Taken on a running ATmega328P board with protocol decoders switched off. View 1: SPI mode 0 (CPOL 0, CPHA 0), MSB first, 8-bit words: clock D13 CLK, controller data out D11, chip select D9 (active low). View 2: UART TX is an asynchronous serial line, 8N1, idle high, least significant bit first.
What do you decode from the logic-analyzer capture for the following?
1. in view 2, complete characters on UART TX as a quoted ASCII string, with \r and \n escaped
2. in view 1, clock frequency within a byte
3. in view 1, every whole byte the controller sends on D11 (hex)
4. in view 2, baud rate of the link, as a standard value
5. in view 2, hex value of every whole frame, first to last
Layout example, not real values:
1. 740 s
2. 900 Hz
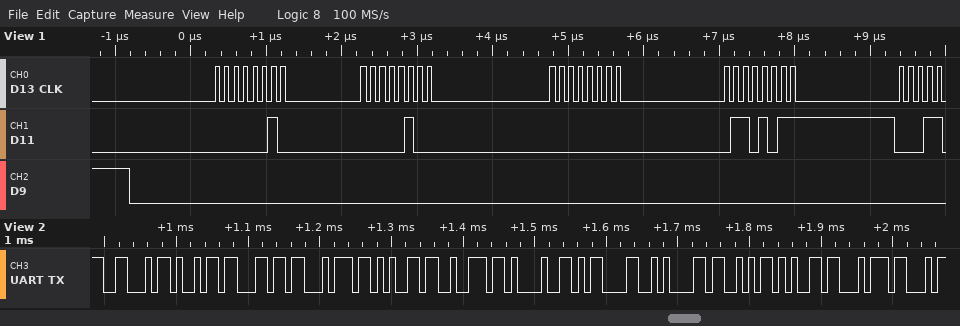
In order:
1. "Filter!\r\nSet"
2. 8 MHz
3. 02 04 00 6B
4. 115200 baud
5. 0x46 0x69 0x6C 0x74 0x65 0x72 0x21 0x0D 0x0A 0x53 0x65 0x74
